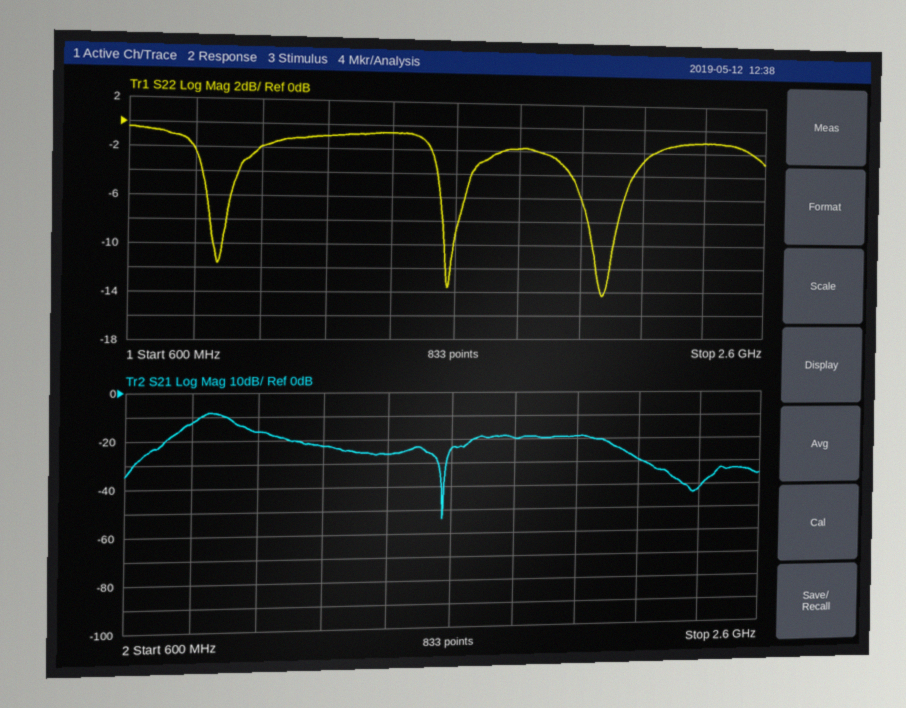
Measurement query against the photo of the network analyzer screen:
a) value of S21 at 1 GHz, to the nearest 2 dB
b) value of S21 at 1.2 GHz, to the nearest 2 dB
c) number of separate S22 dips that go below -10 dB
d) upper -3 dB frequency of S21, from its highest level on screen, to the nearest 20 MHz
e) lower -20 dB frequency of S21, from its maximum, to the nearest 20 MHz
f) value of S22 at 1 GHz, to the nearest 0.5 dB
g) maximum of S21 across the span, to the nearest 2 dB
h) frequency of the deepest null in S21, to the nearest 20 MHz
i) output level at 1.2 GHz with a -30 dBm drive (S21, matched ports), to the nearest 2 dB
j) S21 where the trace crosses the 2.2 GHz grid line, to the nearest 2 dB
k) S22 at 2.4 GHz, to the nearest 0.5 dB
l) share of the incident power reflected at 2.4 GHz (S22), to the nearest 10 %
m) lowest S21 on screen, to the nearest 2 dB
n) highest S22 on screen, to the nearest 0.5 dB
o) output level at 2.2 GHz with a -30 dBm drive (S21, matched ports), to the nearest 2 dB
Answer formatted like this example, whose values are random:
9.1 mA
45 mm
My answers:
-16 dB
-22 dB
3
920 MHz
640 MHz
-2.0 dB
-8 dB
1.58 GHz
-52 dBm
-30 dB
-1.0 dB
80 %
-54 dB
-0.5 dB
-60 dBm
